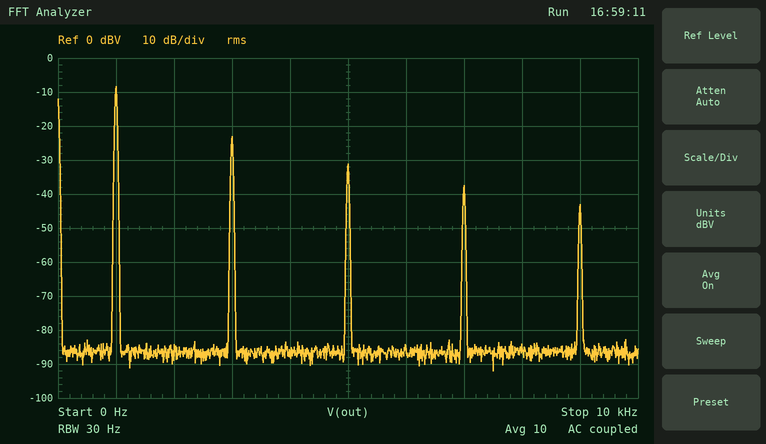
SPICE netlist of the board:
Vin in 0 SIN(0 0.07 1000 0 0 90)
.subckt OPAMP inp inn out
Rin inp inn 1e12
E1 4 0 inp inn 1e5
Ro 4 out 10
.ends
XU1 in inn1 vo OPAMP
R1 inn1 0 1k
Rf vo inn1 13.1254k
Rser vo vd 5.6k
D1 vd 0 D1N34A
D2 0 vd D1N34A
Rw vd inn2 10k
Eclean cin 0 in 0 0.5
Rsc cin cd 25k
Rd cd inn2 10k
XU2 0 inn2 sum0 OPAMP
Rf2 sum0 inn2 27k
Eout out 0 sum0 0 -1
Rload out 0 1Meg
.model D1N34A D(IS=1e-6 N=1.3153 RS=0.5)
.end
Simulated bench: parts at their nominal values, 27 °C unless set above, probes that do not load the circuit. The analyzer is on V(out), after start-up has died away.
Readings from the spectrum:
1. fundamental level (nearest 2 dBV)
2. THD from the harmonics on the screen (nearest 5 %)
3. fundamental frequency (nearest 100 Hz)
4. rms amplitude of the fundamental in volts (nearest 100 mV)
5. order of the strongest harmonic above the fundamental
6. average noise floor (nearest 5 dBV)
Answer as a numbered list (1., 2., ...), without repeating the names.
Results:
1. -8 dBV
2. 20 %
3. 1.0 kHz
4. 400 mV
5. 3
6. -85 dBV
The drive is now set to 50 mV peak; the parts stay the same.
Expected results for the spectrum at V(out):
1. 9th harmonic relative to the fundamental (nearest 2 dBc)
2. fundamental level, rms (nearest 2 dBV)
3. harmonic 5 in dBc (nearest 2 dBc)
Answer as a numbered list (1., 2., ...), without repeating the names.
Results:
1. -40 dBc
2. -10 dBV
3. -26 dBc
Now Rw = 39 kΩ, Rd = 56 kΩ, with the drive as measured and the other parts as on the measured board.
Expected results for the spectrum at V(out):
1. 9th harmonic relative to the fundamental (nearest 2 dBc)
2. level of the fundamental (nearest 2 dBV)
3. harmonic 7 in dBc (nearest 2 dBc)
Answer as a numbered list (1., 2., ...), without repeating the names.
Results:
1. -32 dBc
2. -20 dBV
3. -28 dBc
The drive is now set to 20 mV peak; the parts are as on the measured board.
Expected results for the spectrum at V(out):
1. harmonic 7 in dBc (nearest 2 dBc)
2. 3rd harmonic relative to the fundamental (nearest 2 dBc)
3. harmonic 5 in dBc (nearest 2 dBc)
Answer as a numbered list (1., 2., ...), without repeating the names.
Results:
1. -54 dBc
2. -22 dBc
3. -38 dBc
